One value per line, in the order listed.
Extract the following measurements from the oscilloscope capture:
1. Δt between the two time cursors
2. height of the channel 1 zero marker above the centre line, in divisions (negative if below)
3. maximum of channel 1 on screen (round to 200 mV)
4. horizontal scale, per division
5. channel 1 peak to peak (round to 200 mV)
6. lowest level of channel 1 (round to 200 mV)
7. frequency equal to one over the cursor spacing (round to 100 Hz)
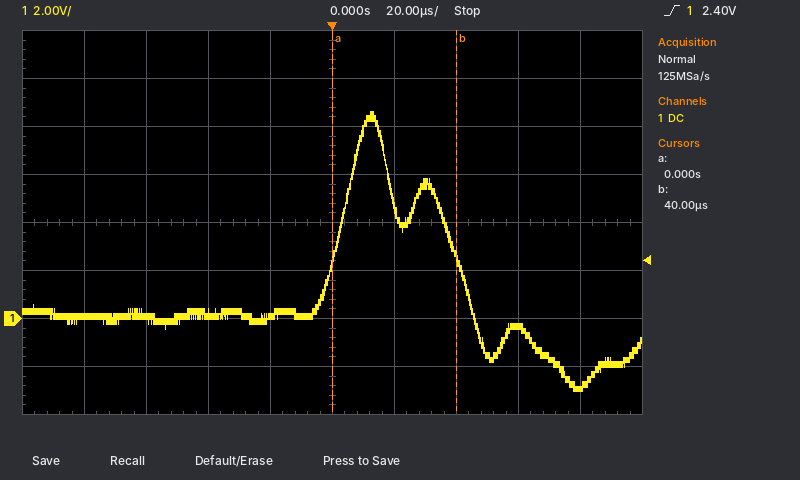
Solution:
40 µs
-2.0 div
8.6 V
20 µs
11.6 V
-3.0 V
25.0 kHz
